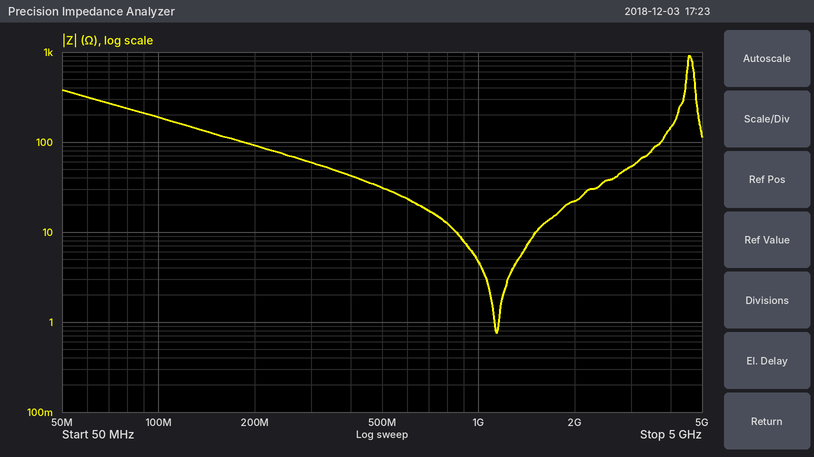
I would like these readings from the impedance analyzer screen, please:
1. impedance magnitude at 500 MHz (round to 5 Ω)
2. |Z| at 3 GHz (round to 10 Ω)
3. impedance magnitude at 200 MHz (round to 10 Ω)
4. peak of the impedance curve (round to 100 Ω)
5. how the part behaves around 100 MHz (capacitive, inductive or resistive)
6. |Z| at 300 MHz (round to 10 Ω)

30 Ω
50 Ω
90 Ω
900 Ω
capacitive
60 Ω
